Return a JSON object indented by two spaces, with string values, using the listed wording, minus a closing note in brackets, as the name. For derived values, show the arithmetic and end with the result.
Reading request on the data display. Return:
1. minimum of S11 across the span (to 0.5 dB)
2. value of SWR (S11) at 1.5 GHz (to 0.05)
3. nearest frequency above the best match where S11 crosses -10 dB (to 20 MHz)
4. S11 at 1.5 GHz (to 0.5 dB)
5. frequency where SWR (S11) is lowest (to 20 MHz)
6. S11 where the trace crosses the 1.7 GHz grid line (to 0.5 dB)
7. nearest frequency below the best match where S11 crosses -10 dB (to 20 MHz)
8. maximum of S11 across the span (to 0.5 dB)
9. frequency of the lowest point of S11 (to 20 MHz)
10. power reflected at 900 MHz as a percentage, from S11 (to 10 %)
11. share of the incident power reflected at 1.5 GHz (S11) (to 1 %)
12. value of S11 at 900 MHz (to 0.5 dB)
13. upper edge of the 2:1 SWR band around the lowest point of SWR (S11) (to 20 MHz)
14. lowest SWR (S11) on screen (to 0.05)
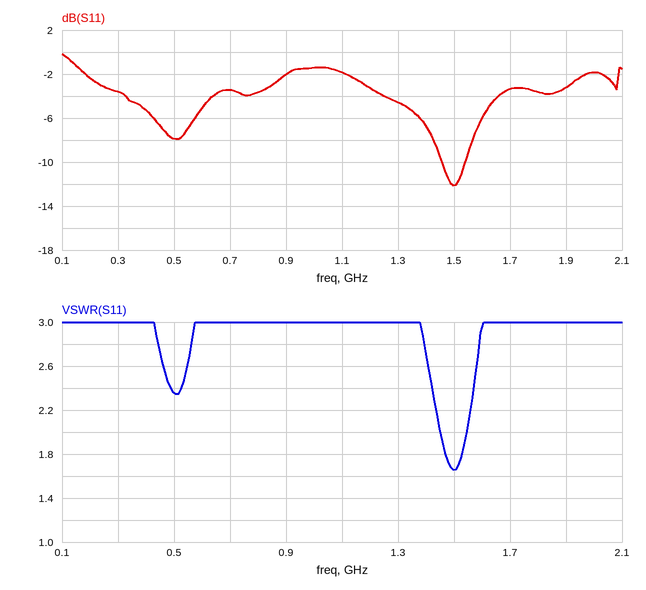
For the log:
{
  "minimum of S11 across the span": "-12.0 dB",
  "value of SWR (S11) at 1.5 GHz": "1.65",
  "nearest frequency above the best match where S11 crosses -10 dB": "1.54 GHz",
  "S11 at 1.5 GHz": "-12.0 dB",
  "frequency where SWR (S11) is lowest": "1.50 GHz",
  "S11 where the trace crosses the 1.7 GHz grid line": "-3.5 dB",
  "nearest frequency below the best match where S11 crosses -10 dB": "1.46 GHz",
  "maximum of S11 across the span": "0.0 dB",
  "frequency of the lowest point of S11": "1.50 GHz",
  "power reflected at 900 MHz as a percentage, from S11": "10^(-2/10) ≈ 63.1 %, so 60 % to the nearest 10 %",
  "share of the incident power reflected at 1.5 GHz (S11)": "10^(-12/10) ≈ 6 %",
  "value of S11 at 900 MHz": "-2.0 dB",
  "upper edge of the 2:1 SWR band around the lowest point of SWR (S11)": "1.54 GHz",
  "lowest SWR (S11) on screen": "1.65"
}
